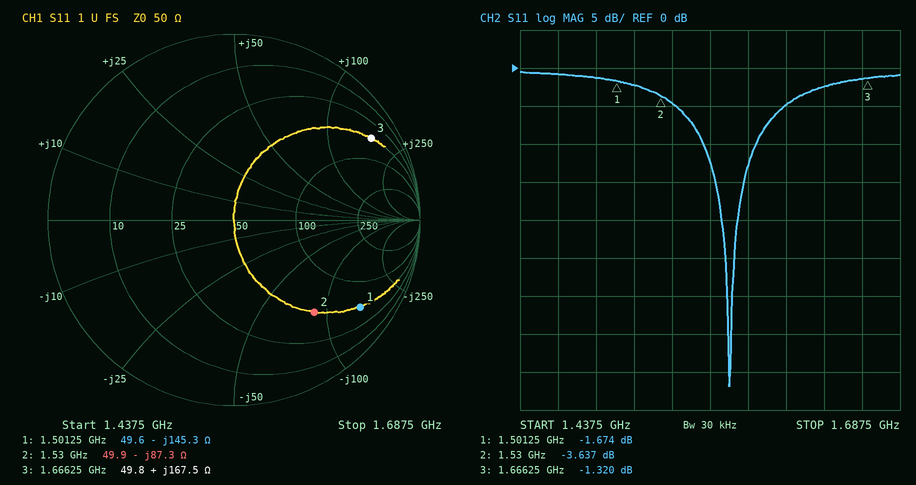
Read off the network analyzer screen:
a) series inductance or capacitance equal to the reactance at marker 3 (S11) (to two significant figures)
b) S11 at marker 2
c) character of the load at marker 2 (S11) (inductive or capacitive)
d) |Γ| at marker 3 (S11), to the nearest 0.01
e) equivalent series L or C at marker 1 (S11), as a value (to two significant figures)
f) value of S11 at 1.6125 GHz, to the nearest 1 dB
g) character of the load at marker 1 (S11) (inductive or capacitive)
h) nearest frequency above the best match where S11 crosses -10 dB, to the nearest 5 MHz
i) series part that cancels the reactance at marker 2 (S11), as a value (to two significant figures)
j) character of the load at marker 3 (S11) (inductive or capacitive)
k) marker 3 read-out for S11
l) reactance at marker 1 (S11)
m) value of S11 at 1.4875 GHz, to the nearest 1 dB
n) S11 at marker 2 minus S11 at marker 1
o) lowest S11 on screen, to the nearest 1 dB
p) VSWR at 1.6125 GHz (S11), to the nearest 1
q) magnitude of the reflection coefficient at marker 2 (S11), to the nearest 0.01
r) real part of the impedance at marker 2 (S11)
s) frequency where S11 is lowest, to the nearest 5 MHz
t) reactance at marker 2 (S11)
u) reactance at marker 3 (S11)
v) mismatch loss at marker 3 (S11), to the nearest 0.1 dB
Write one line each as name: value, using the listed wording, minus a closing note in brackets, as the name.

series inductance or capacitance equal to the reactance at marker 3 (S11): 16 nH
S11 at marker 2: -3.637 dB
character of the load at marker 2 (S11): capacitive
|Γ| at marker 3 (S11), to the nearest 0.01: 0.86
equivalent series L or C at marker 1 (S11), as a value: 730 fF
value of S11 at 1.6125 GHz, to the nearest 1 dB: -5 dB
character of the load at marker 1 (S11): capacitive
nearest frequency above the best match where S11 crosses -10 dB, to the nearest 5 MHz: 1.595 GHz
series part that cancels the reactance at marker 2 (S11), as a value: 9.1 nH
character of the load at marker 3 (S11): inductive
marker 3 read-out for S11: -1.320 dB
reactance at marker 1: -145.3 Ω
value of S11 at 1.4875 GHz, to the nearest 1 dB: -1 dB
S11 at marker 2 minus S11 at marker 1: -1.963 dB
lowest S11 on screen, to the nearest 1 dB: -42 dB
VSWR at 1.6125 GHz (S11), to the nearest 1: 4
magnitude of the reflection coefficient at marker 2 (S11), to the nearest 0.01: 0.66
real part of the impedance at marker 2: 49.9 Ω
frequency where S11 is lowest, to the nearest 5 MHz: 1.575 GHz
reactance at marker 2: -87.3 Ω
reactance at marker 3: +167.5 Ω
mismatch loss at marker 3 (S11), to the nearest 0.1 dB: 5.8 dB
